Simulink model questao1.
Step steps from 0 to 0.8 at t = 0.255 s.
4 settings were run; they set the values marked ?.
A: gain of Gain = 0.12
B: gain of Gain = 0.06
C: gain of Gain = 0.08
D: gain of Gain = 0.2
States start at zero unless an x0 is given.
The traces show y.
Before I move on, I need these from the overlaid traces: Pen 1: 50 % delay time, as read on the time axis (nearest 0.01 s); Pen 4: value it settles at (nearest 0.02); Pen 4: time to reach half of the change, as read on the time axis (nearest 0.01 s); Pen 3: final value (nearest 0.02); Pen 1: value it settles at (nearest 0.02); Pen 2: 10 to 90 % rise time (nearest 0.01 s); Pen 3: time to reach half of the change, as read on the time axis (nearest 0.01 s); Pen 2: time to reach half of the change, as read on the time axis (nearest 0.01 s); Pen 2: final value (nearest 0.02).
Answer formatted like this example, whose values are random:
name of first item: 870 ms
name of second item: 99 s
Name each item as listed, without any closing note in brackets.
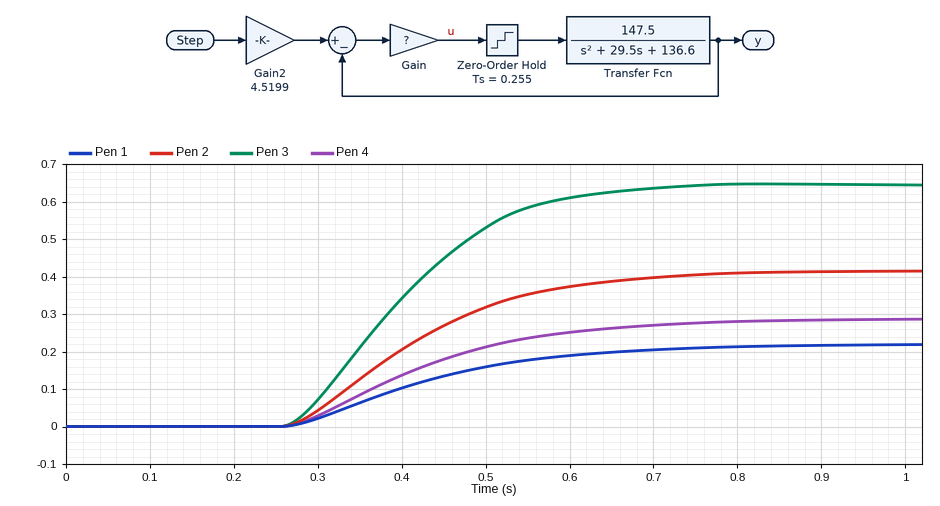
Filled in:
Pen 1: 50 % delay time, as read on the time axis: 0.41 s
Pen 4: value it settles at: 0.28
Pen 4: time to reach half of the change, as read on the time axis: 0.41 s
Pen 3: final value: 0.64
Pen 1: value it settles at: 0.22
Pen 2: 10 to 90 % rise time: 0.30 s
Pen 3: time to reach half of the change, as read on the time axis: 0.39 s
Pen 2: time to reach half of the change, as read on the time axis: 0.40 s
Pen 2: final value: 0.42
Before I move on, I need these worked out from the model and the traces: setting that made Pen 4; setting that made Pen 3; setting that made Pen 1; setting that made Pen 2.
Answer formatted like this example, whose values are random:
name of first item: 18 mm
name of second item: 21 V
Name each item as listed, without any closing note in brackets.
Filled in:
setting that made Pen 4: C
setting that made Pen 3: D
setting that made Pen 1: B
setting that made Pen 2: A
